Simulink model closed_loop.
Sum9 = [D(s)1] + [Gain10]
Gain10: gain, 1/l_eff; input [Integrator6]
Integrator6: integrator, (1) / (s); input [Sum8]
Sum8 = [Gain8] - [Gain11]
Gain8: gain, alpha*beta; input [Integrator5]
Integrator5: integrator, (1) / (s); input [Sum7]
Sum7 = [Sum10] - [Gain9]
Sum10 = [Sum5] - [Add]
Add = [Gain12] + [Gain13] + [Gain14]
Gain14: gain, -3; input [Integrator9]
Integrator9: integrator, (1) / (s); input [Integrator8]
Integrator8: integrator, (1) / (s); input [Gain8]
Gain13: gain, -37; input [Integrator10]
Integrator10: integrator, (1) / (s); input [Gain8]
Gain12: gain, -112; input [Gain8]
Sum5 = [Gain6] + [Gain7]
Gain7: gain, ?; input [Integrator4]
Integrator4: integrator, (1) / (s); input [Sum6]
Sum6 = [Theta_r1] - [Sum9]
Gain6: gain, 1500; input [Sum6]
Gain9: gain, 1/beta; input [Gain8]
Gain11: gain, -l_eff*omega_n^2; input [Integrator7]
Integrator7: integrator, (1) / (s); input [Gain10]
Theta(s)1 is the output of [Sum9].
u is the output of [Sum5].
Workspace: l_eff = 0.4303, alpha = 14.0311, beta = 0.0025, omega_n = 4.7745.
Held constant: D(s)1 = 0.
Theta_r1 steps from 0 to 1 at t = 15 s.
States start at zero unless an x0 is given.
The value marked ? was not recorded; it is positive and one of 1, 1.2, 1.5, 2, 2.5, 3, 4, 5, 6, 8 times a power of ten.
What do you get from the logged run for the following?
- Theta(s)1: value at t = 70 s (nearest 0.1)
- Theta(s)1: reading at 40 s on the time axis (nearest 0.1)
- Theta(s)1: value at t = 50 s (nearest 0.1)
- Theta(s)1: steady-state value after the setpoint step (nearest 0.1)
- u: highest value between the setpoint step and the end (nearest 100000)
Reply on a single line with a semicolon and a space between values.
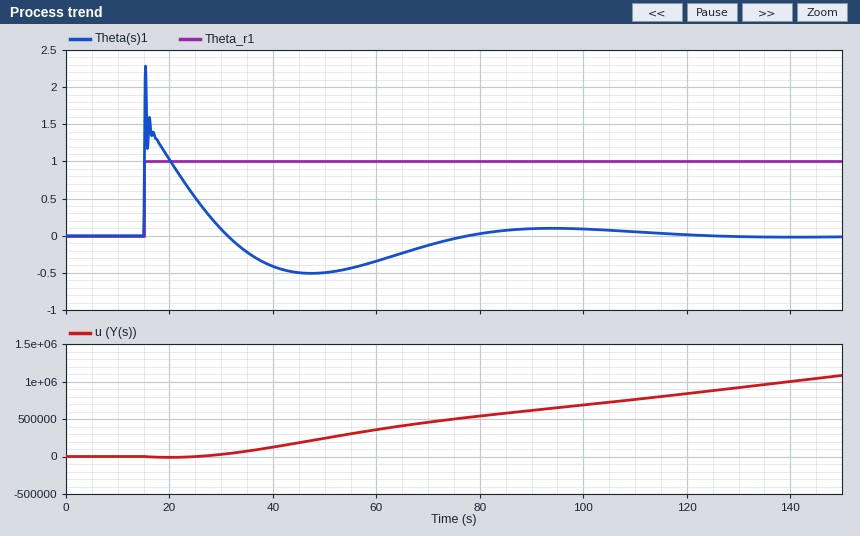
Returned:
-0.1; -0.4; -0.5; 0.0; 1100000
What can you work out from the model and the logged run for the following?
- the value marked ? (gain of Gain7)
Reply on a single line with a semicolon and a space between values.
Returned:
8000
